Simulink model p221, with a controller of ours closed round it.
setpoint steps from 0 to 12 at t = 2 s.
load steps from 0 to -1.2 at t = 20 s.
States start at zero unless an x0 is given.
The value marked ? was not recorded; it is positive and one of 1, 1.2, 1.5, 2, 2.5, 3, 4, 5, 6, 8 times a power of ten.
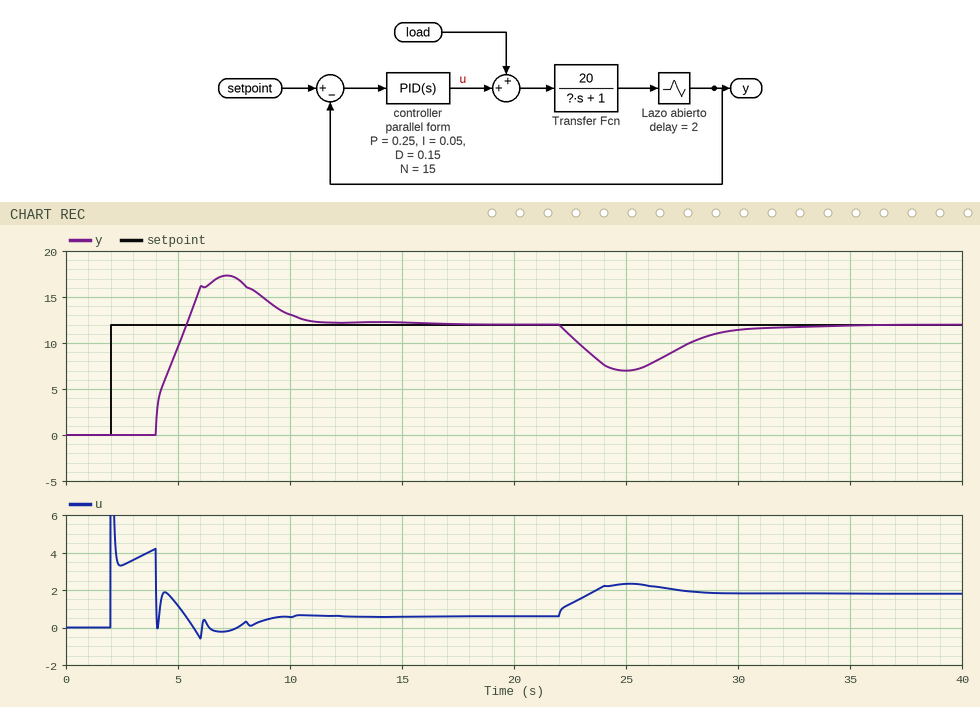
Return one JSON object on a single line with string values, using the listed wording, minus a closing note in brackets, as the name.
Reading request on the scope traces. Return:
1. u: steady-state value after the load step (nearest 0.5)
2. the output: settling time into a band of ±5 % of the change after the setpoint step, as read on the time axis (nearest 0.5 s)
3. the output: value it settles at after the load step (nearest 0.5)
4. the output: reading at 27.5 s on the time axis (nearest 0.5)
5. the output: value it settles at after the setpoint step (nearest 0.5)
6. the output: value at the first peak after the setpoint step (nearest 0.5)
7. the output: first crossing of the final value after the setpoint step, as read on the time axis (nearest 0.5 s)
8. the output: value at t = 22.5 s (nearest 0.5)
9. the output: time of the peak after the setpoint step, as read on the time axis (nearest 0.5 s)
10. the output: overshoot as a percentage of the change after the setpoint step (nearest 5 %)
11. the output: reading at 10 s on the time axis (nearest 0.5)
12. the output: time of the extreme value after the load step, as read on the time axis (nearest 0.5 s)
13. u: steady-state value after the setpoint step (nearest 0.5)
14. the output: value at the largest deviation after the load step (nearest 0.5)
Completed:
{"u: steady-state value after the load step": "2.0", "the output: settling time into a band of ±5 % of the change after the setpoint step, as read on the time axis": "10.5 s", "the output: value it settles at after the load step": "12.0", "the output: reading at 27.5 s on the time axis": "9.5", "the output: value it settles at after the setpoint step": "12.0", "the output: value at the first peak after the setpoint step": "17.5", "the output: first crossing of the final value after the setpoint step, as read on the time axis": "5.5 s", "the output: value at t = 22.5 s": "11.0", "the output: time of the peak after the setpoint step, as read on the time axis": "7.0 s", "the output: overshoot as a percentage of the change after the setpoint step": "45 %", "the output: reading at 10 s on the time axis": "13.0", "the output: time of the extreme value after the load step, as read on the time axis": "25.0 s", "u: steady-state value after the setpoint step": "0.5", "the output: value at the largest deviation after the load step": "7.0"}
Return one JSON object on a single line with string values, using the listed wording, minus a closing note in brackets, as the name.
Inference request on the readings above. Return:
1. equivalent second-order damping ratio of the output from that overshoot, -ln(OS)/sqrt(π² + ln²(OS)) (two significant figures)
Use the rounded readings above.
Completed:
{"equivalent second-order damping ratio of the output from that overshoot, -ln(OS)/sqrt(π² + ln²(OS))": "0.25"}
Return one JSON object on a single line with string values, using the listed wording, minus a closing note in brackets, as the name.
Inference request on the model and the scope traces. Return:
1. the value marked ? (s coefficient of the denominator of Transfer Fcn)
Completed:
{"the value marked ?": "10"}
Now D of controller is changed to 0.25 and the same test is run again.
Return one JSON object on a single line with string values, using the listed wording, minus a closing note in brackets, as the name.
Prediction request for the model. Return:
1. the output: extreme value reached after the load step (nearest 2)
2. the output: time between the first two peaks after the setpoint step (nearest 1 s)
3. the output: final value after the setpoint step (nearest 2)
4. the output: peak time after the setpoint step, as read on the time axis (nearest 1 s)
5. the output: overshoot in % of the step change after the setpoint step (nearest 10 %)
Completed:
{"the output: extreme value reached after the load step": "8", "the output: time between the first two peaks after the setpoint step": "5 s", "the output: final value after the setpoint step": "12", "the output: peak time after the setpoint step, as read on the time axis": "6 s", "the output: overshoot in % of the step change after the setpoint step": "50 %"}
